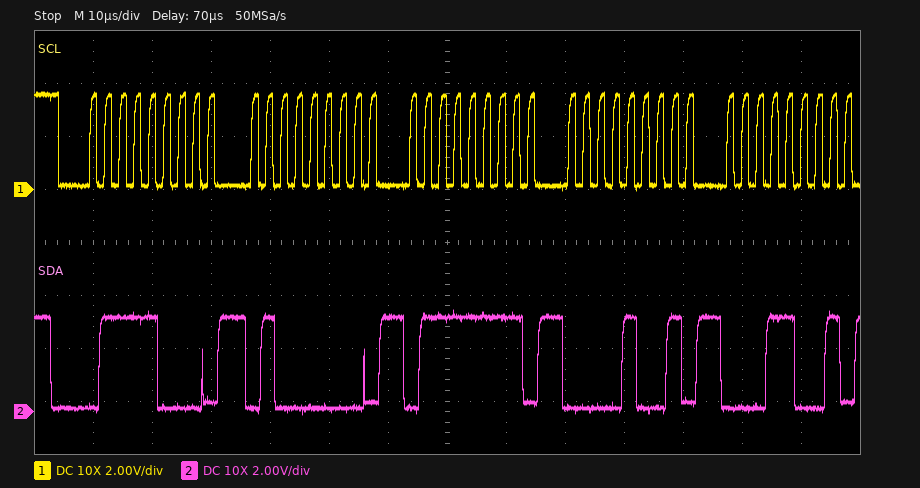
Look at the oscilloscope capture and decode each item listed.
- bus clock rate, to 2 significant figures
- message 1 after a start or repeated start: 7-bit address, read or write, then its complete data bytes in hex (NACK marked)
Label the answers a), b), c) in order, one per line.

a) 400 kHz
b) 0x3C write: 40 7F 09 19
